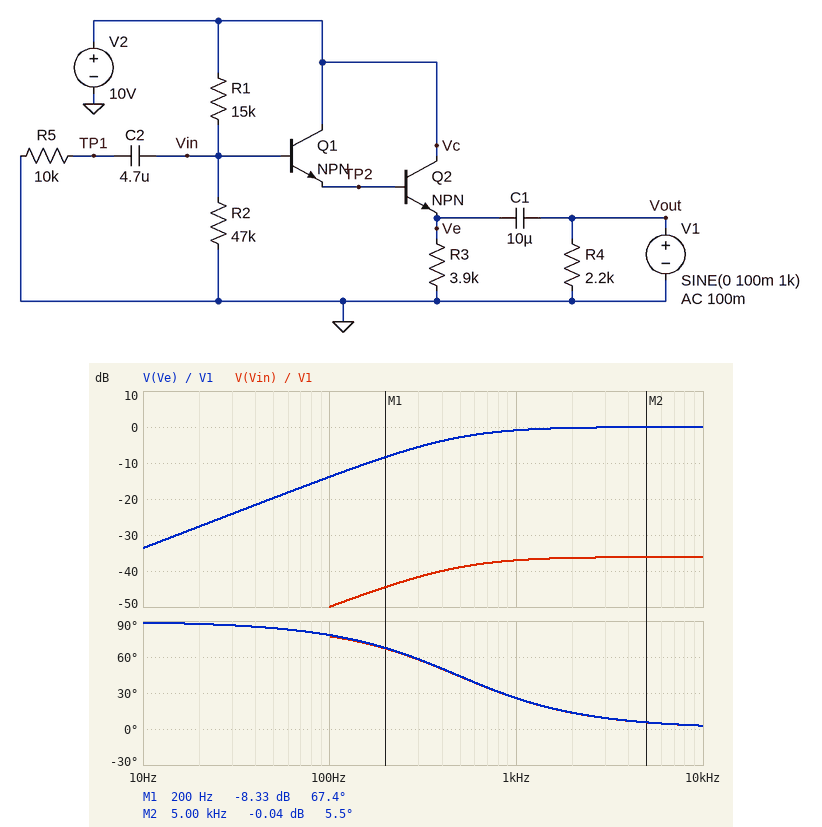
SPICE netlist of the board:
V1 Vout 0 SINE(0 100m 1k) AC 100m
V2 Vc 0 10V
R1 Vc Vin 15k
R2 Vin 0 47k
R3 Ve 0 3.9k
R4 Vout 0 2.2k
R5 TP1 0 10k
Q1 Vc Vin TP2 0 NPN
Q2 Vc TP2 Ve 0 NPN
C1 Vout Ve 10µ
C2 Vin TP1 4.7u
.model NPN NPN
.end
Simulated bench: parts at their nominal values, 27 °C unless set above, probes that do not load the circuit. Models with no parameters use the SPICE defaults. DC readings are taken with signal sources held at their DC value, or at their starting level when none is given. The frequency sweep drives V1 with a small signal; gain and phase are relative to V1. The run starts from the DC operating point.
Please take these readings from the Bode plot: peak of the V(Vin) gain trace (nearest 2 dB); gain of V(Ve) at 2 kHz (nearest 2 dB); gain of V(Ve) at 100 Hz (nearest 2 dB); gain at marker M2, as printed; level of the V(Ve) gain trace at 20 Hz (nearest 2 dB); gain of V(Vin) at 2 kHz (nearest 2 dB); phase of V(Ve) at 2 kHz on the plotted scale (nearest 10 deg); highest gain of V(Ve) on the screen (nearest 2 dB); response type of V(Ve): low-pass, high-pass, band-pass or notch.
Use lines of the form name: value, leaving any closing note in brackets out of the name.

peak of the V(Vin) gain trace: -36 dB
gain of V(Ve) at 2 kHz: 0 dB
gain of V(Ve) at 100 Hz: -14 dB
gain at marker M2, as printed: -0.04 dB
level of the V(Ve) gain trace at 20 Hz: -28 dB
gain of V(Vin) at 2 kHz: -36 dB
phase of V(Ve) at 2 kHz on the plotted scale: 10 deg
highest gain of V(Ve) on the screen: 0 dB
response type of V(Ve): low-pass, high-pass, band-pass or notch: high-pass
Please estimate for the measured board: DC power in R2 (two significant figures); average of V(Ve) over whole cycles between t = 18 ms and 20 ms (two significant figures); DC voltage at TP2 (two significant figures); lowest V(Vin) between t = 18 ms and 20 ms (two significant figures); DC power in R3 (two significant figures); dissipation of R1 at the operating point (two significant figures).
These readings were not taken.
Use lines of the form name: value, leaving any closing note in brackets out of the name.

DC power in R2: 1.2 mW
average of V(Ve) over whole cycles between t = 18 ms and 20 ms: 6.2 V
DC voltage at TP2: 6.9 V
lowest V(Vin) between t = 18 ms and 20 ms: 7.6 V
DC power in R3: 9.6 mW
dissipation of R1 at the operating point: 390 µW
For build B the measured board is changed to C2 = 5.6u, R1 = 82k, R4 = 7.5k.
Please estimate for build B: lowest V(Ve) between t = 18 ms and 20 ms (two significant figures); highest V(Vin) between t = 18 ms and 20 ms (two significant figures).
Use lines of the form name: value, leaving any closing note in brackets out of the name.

lowest V(Ve) between t = 18 ms and 20 ms: 2.2 V
highest V(Vin) between t = 18 ms and 20 ms: 3.6 V
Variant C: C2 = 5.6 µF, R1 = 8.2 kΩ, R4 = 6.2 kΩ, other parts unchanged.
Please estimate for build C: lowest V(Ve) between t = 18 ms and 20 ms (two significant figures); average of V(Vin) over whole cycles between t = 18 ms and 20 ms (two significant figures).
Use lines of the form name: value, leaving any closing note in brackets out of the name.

lowest V(Ve) between t = 18 ms and 20 ms: 7.0 V
average of V(Vin) over whole cycles between t = 18 ms and 20 ms: 8.5 V
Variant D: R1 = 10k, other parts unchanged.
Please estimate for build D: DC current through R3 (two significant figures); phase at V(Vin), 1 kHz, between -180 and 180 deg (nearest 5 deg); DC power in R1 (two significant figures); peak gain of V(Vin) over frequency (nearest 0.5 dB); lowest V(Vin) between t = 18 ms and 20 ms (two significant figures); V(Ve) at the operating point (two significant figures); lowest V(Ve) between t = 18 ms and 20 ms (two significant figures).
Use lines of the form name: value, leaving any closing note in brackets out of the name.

DC current through R3: 1.7 mA
phase at V(Vin), 1 kHz, between -180 and 180 deg: 30 deg
DC power in R1: 310 µW
peak gain of V(Vin) over frequency: -36.5 dB
lowest V(Vin) between t = 18 ms and 20 ms: 8.2 V
V(Ve) at the operating point: 6.8 V
lowest V(Ve) between t = 18 ms and 20 ms: 6.7 V
